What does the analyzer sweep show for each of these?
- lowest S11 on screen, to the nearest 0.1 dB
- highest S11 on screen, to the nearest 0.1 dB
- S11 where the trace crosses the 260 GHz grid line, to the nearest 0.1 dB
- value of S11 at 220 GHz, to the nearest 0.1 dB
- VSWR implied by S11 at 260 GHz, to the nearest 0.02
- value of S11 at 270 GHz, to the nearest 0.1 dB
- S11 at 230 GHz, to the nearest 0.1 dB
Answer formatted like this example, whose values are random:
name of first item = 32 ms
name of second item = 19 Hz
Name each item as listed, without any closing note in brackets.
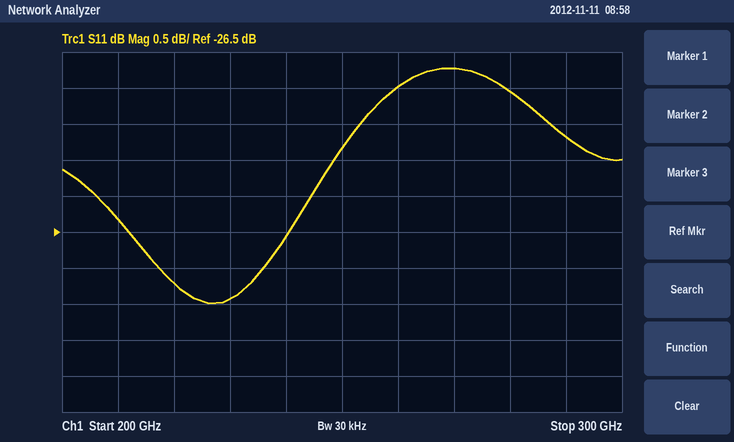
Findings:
lowest S11 on screen, to the nearest 0.1 dB = -27.5 dB
highest S11 on screen, to the nearest 0.1 dB = -24.2 dB
S11 where the trace crosses the 260 GHz grid line, to the nearest 0.1 dB = -24.5 dB
value of S11 at 220 GHz, to the nearest 0.1 dB = -27.2 dB
VSWR implied by S11 at 260 GHz, to the nearest 0.02 = 1.12
value of S11 at 270 GHz, to the nearest 0.1 dB = -24.2 dB
S11 at 230 GHz, to the nearest 0.1 dB = -27.4 dB
